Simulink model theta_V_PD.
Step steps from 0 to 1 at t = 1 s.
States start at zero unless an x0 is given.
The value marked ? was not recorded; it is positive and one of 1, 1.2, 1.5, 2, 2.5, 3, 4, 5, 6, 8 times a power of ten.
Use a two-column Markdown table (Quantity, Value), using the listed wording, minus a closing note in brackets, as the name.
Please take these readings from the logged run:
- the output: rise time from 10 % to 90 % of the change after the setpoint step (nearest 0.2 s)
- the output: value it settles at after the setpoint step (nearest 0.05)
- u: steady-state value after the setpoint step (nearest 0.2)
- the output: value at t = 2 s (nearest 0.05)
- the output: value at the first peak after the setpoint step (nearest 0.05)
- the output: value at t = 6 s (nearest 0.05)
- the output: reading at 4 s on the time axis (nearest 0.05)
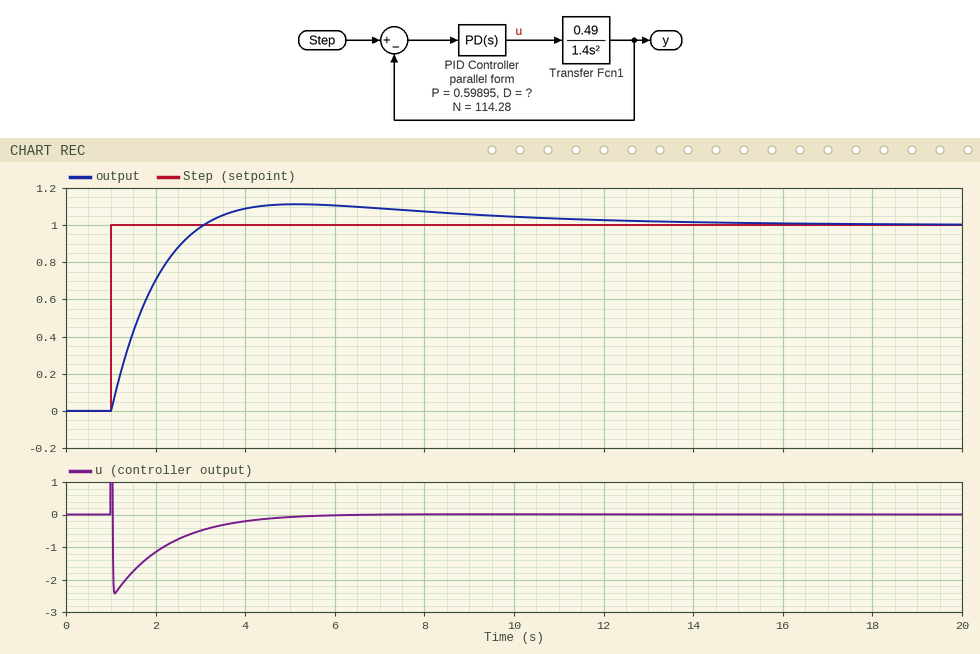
| Quantity | Value |
|---|---|
| the output: rise time from 10 % to 90 % of the change after the setpoint step | 1.4 s |
| the output: value it settles at after the setpoint step | 1.00 |
| u: steady-state value after the setpoint step | 0.0 |
| the output: value at t = 2 s | 0.70 |
| the output: value at the first peak after the setpoint step | 1.10 |
| the output: value at t = 6 s | 1.10 |
| the output: reading at 4 s on the time axis | 1.10 |
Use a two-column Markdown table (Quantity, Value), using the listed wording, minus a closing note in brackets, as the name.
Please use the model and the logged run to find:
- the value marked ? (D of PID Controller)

| Quantity | Value |
|---|---|
| the value marked ? | 3 |
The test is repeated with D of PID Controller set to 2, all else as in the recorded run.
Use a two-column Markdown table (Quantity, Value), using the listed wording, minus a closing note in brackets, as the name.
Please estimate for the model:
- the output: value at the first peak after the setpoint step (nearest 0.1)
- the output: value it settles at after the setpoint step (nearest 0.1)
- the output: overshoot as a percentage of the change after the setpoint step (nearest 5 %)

| Quantity | Value |
|---|---|
| the output: value at the first peak after the setpoint step | 1.2 |
| the output: value it settles at after the setpoint step | 1.0 |
| the output: overshoot as a percentage of the change after the setpoint step | 20 % |
